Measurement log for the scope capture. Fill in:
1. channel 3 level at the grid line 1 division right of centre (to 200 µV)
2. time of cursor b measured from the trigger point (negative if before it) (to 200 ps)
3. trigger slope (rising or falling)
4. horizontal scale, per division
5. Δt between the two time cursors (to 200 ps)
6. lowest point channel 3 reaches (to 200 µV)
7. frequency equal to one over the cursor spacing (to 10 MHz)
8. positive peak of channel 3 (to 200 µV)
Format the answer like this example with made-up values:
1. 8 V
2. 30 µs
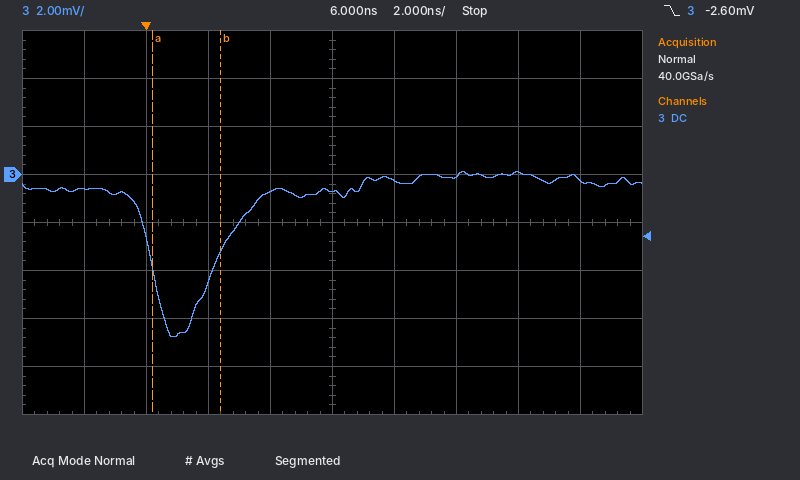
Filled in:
1. -200 µV
2. +2.4 ns
3. falling
4. 2 ns
5. 2.2 ns
6. -6.8 mV
7. 450 MHz
8. 200 µV
